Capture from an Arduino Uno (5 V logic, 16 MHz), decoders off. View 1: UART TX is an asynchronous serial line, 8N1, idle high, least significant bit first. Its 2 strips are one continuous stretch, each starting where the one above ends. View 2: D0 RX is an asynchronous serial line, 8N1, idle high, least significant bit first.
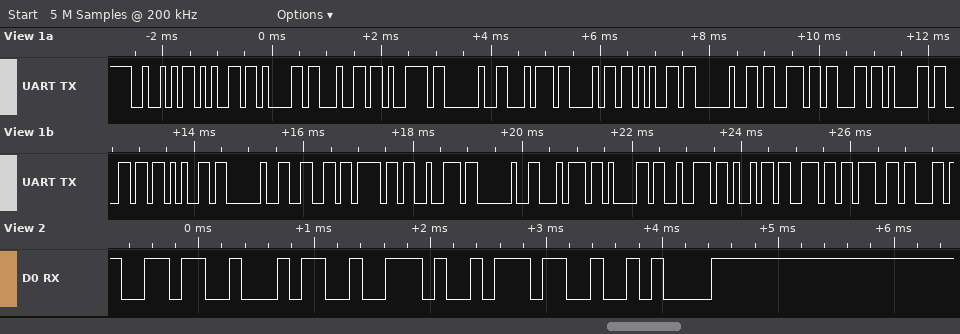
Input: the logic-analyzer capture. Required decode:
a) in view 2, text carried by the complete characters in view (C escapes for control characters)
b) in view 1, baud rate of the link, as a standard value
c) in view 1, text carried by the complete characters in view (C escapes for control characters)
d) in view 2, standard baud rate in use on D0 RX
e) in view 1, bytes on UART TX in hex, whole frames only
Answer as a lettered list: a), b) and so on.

a) "64.7\n"
b) 9600 baud
c) "Ready the scale for taring"
d) 9600 baud
e) 0x52 0x65 0x61 0x64 0x79 0x20 0x74 0x68 0x65 0x20 0x73 0x63 0x61 0x6C 0x65 0x20 0x66 0x6F 0x72 0x20 0x74 0x61 0x72 0x69 0x6E 0x67
